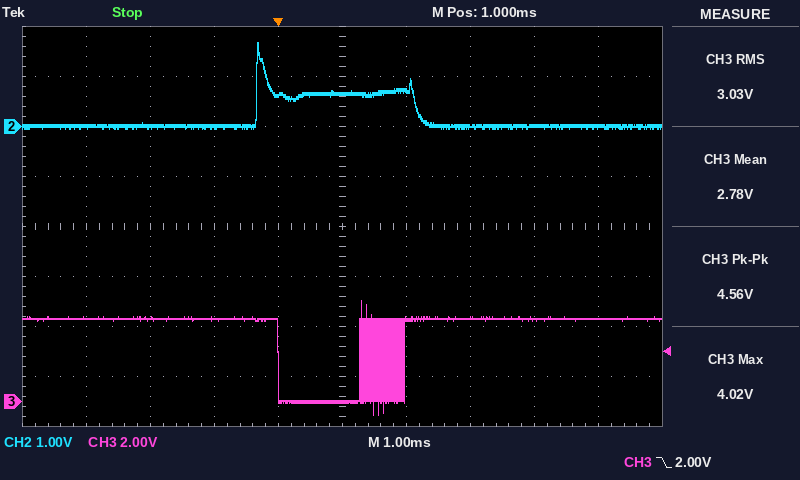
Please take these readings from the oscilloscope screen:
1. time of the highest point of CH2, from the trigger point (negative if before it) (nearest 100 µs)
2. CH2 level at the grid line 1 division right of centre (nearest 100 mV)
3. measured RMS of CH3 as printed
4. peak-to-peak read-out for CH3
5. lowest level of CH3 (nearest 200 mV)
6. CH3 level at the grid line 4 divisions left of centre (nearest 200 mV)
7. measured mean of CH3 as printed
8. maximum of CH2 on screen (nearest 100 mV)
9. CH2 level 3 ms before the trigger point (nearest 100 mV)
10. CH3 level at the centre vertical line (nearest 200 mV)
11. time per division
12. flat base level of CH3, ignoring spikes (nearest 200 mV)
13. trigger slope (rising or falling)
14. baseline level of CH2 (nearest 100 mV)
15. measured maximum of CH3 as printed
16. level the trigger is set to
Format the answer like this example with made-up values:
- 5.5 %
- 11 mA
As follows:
- -300 µs
- 700 mV
- 3.03 V
- 4.56 V
- -600 mV
- 3.4 V
- 2.78 V
- 1.7 V
- 0.0 V
- 0.0 V
- 1 ms
- 0.0 V
- falling
- 0.0 V
- 4.02 V
- 2.00 V
